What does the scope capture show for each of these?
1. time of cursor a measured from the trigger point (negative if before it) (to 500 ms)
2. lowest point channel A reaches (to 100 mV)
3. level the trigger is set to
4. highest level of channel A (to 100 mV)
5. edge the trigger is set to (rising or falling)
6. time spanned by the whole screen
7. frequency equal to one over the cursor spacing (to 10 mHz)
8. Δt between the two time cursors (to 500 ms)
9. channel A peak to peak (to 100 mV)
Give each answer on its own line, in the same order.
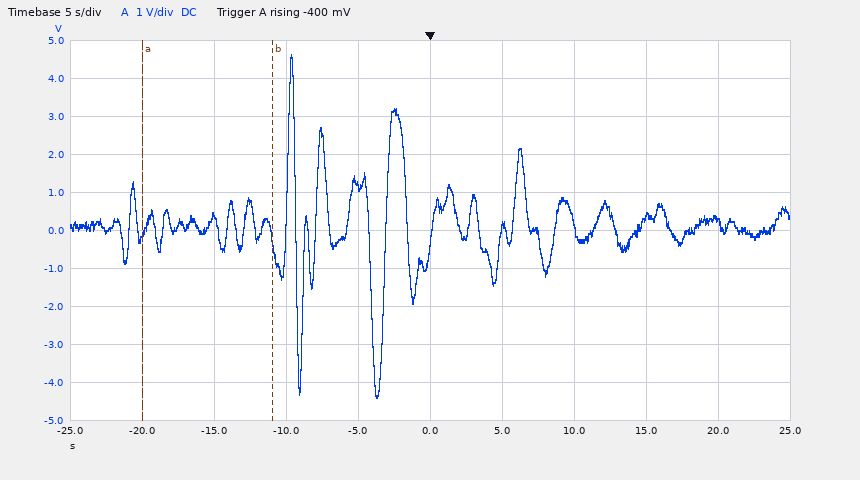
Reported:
-20.0 s
-4.4 V
-400 mV
4.6 V
rising
50 s
110 mHz
9.0 s
9.0 V
